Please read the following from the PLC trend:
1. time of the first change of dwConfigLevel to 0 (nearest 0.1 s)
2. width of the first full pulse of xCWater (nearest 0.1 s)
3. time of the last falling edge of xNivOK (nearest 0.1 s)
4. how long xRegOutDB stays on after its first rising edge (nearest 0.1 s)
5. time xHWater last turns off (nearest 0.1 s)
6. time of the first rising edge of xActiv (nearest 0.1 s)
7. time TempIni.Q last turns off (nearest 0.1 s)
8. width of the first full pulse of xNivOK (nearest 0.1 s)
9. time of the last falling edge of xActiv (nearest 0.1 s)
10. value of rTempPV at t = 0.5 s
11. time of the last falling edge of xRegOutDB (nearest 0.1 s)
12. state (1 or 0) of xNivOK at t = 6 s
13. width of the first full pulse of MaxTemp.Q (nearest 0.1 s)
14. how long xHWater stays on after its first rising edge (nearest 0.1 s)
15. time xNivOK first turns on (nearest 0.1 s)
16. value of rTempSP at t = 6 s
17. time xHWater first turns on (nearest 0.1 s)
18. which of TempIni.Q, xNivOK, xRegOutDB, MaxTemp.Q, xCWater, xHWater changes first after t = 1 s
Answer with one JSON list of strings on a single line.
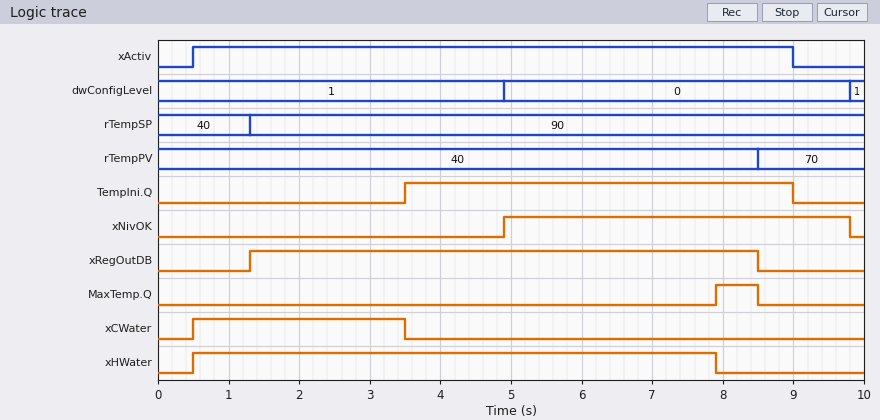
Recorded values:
["4.9 s", "3.0 s", "9.8 s", "7.2 s", "7.9 s", "0.5 s", "9.0 s", "4.9 s", "9.0 s", "40", "8.5 s", "1", "0.6 s", "7.4 s", "4.9 s", "90", "0.5 s", "xRegOutDB"]
